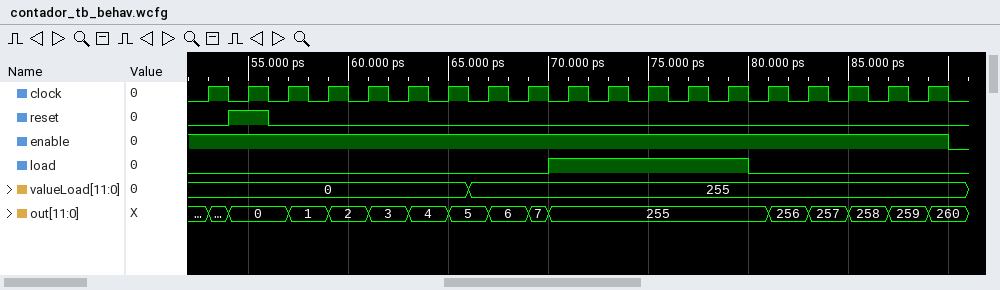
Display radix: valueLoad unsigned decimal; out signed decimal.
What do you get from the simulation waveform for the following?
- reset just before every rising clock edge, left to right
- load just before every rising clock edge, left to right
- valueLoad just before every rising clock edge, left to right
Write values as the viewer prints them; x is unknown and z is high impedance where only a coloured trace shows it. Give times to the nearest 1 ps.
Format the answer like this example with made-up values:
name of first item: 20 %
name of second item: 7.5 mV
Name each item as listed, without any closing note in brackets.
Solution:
reset just before every rising clock edge, left to right: 0 1 0 0 0 0 0 0 0 0 0 0 0 0 0 0 0 0 0
load just before every rising clock edge, left to right: 0 0 0 0 0 0 0 0 0 1 1 1 1 1 0 0 0 0 0
valueLoad just before every rising clock edge, left to right: 0, 0, 0, 0, 0, 0, 0, 255, 255, 255, 255, 255, 255, 255, 255, 255, 255, 255, 255
